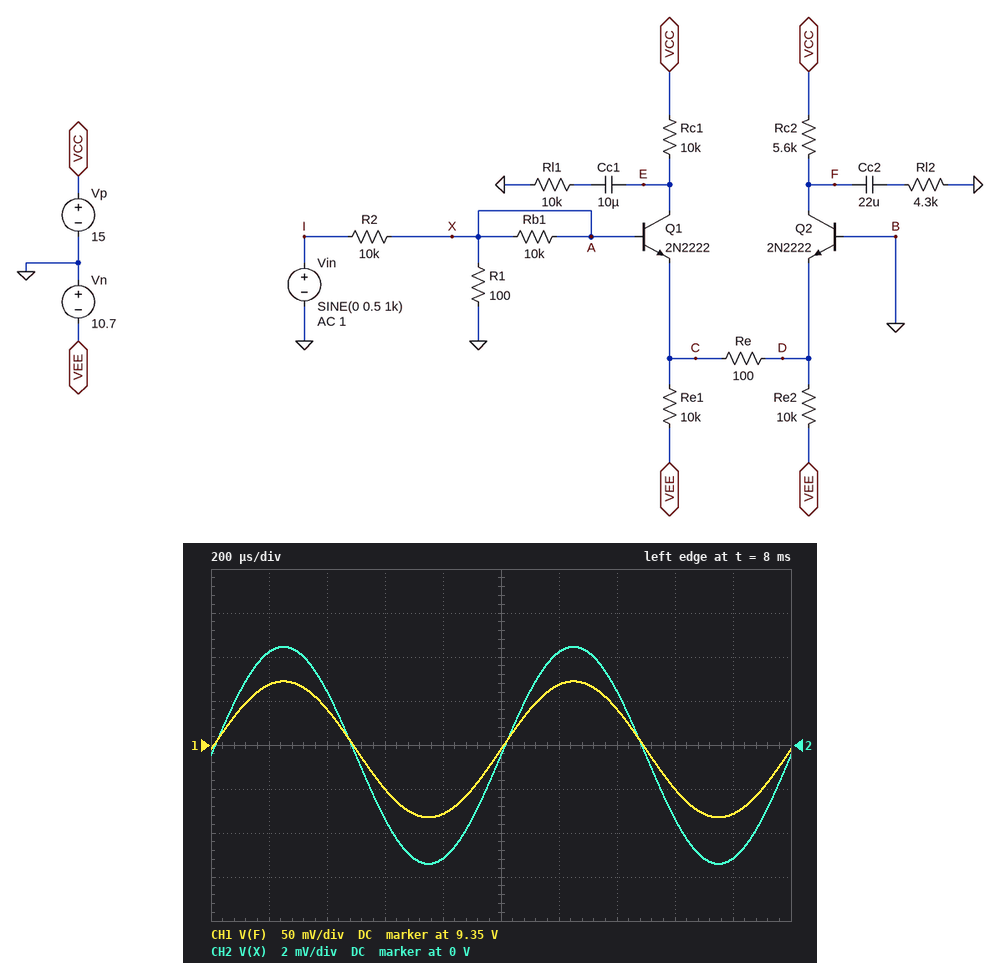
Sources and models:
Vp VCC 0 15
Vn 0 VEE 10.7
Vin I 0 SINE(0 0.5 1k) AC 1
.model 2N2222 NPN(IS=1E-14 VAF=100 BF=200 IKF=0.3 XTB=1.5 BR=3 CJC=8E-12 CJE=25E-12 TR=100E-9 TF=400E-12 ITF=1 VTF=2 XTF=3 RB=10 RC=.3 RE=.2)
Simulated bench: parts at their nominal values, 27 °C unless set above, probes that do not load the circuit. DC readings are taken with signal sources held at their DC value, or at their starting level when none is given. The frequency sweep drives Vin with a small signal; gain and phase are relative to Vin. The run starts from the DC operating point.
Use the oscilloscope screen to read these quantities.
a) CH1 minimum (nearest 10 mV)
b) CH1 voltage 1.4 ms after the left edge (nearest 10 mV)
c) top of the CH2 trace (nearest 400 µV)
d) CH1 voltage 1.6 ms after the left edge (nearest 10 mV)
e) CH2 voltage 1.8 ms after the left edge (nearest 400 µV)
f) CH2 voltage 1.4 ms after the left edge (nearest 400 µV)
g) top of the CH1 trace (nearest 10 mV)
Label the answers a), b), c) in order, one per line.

a) 9.27 V
b) 9.39 V
c) 4.4 mV
d) 9.30 V
e) -5.2 mV
f) 2.4 mV
g) 9.42 V
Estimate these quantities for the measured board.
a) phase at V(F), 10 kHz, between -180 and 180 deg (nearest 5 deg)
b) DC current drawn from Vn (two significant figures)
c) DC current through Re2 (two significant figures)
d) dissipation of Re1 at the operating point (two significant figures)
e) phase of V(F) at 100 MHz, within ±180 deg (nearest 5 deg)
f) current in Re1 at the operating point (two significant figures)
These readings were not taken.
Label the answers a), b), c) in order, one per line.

a) 0 deg
b) 2.0 mA
c) 1.0 mA
d) 10 mW
e) -115 deg
f) 1.0 mA
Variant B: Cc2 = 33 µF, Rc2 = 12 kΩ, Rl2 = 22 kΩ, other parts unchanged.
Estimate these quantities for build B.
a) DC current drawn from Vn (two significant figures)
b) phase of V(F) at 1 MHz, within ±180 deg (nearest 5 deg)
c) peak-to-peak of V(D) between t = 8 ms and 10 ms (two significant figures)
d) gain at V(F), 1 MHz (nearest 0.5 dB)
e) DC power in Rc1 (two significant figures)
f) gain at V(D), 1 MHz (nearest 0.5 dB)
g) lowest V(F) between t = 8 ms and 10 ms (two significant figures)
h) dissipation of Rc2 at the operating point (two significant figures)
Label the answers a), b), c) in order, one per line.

a) 2.0 mA
b) -20 deg
c) 1.8 mV
d) -6.5 dB
e) 10 mW
f) -55.0 dB
g) 2.8 V
h) 12 mW
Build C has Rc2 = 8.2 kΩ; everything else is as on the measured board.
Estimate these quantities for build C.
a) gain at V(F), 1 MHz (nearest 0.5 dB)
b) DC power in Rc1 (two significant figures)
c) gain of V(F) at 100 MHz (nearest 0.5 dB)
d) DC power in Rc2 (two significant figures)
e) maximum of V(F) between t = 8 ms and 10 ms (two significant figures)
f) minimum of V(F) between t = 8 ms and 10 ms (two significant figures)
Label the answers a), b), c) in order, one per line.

a) -15.0 dB
b) 9.9 mW
c) -38.5 dB
d) 8.3 mW
e) 6.8 V
f) 6.7 V
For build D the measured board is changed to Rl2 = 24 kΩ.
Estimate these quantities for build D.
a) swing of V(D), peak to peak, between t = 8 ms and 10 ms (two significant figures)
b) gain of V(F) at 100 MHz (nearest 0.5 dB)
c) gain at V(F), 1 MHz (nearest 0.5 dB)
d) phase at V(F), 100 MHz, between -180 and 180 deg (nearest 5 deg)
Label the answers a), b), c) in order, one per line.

a) 1.7 mV
b) -37.5 dB
c) -11.0 dB
d) -120 deg
